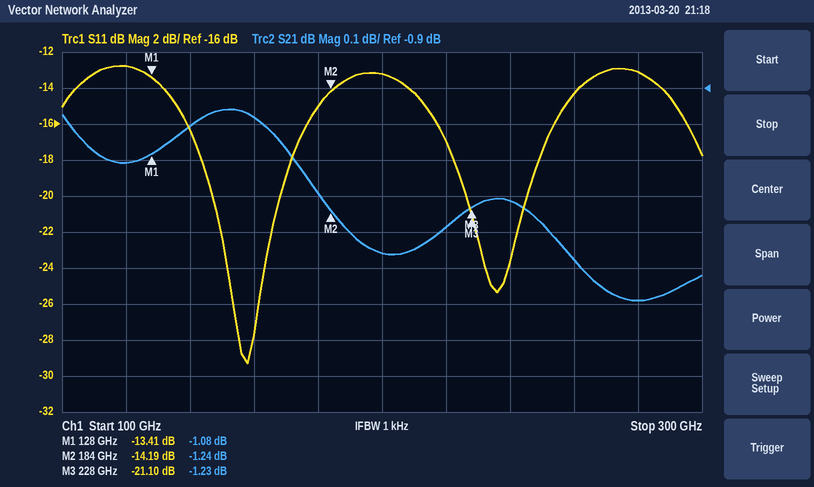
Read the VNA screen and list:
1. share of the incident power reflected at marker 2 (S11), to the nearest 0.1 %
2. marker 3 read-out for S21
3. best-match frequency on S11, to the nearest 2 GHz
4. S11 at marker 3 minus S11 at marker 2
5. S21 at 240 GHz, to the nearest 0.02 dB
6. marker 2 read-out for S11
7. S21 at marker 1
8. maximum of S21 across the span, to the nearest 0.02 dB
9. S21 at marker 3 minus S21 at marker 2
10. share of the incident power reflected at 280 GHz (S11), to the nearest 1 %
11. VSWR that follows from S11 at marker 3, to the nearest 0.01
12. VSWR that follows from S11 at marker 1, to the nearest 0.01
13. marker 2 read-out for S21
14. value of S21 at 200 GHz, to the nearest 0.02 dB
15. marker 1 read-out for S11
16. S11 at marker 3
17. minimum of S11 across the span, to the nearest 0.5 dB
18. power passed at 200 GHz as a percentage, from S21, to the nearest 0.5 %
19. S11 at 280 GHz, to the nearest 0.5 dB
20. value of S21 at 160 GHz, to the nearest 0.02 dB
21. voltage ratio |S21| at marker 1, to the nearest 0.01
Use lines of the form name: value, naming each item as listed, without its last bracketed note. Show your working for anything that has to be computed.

share of the incident power reflected at marker 2 (S11), to the nearest 0.1 %: 10^(-14.19/10) ≈ 3.8 %
marker 3 read-out for S21: -1.23 dB
best-match frequency on S11, to the nearest 2 GHz: 158 GHz
S11 at marker 3 minus S11 at marker 2: -21.1 − (-14.19) = -6.91 dB
S21 at 240 GHz, to the nearest 0.02 dB: -1.22 dB
marker 2 read-out for S11: -14.19 dB
S21 at marker 1: -1.08 dB
maximum of S21 across the span, to the nearest 0.02 dB: -0.96 dB
S21 at marker 3 minus S21 at marker 2: -1.23 − (-1.24) = 0.01 dB
share of the incident power reflected at 280 GHz (S11), to the nearest 1 %: 10^(-13/10) ≈ 5 %
VSWR that follows from S11 at marker 3, to the nearest 0.01: (1 + 0.0881)/(1 − 0.0881) ≈ 1.19
VSWR that follows from S11 at marker 1, to the nearest 0.01: (1 + 0.2136)/(1 − 0.2136) ≈ 1.54
marker 2 read-out for S21: -1.24 dB
value of S21 at 200 GHz, to the nearest 0.02 dB: -1.36 dB
marker 1 read-out for S11: -13.41 dB
S11 at marker 3: -21.10 dB
minimum of S11 across the span, to the nearest 0.5 dB: -29.5 dB
power passed at 200 GHz as a percentage, from S21, to the nearest 0.5 %: 10^(-1.36/10) ≈ 73.1 %, so 73.0 % to the nearest 0.5 %
S11 at 280 GHz, to the nearest 0.5 dB: -13.0 dB
value of S21 at 160 GHz, to the nearest 0.02 dB: -0.98 dB
voltage ratio |S21| at marker 1, to the nearest 0.01: 10^(-1.08/20) ≈ 0.88
